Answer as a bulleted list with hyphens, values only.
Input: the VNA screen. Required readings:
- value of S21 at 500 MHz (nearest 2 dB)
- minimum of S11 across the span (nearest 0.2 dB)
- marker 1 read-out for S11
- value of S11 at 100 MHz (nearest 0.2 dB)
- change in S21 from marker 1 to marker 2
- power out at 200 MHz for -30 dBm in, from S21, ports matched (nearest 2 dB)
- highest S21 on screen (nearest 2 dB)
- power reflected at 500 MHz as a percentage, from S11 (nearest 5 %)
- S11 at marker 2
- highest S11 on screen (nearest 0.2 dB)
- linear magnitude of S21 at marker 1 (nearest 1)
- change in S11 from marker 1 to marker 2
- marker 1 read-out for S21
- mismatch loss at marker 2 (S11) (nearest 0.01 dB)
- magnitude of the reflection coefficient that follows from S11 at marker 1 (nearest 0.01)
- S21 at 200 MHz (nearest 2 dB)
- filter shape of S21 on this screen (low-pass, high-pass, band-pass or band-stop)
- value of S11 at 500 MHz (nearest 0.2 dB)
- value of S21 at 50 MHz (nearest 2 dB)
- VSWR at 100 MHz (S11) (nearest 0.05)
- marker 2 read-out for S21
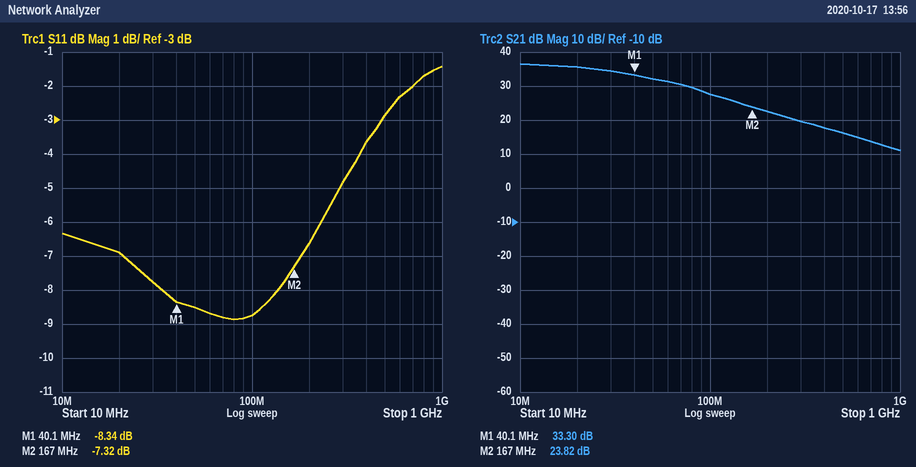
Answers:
- 16 dB
- -8.8 dB
- -8.34 dB
- -8.8 dB
- -9.48 dB
- -8 dBm
- 36 dB
- 50 %
- -7.32 dB
- -1.4 dB
- 46
- 1.02 dB
- 33.30 dB
- 0.89 dB
- 0.38
- 22 dB
- low-pass
- -2.8 dB
- 32 dB
- 2.15
- 23.82 dB
